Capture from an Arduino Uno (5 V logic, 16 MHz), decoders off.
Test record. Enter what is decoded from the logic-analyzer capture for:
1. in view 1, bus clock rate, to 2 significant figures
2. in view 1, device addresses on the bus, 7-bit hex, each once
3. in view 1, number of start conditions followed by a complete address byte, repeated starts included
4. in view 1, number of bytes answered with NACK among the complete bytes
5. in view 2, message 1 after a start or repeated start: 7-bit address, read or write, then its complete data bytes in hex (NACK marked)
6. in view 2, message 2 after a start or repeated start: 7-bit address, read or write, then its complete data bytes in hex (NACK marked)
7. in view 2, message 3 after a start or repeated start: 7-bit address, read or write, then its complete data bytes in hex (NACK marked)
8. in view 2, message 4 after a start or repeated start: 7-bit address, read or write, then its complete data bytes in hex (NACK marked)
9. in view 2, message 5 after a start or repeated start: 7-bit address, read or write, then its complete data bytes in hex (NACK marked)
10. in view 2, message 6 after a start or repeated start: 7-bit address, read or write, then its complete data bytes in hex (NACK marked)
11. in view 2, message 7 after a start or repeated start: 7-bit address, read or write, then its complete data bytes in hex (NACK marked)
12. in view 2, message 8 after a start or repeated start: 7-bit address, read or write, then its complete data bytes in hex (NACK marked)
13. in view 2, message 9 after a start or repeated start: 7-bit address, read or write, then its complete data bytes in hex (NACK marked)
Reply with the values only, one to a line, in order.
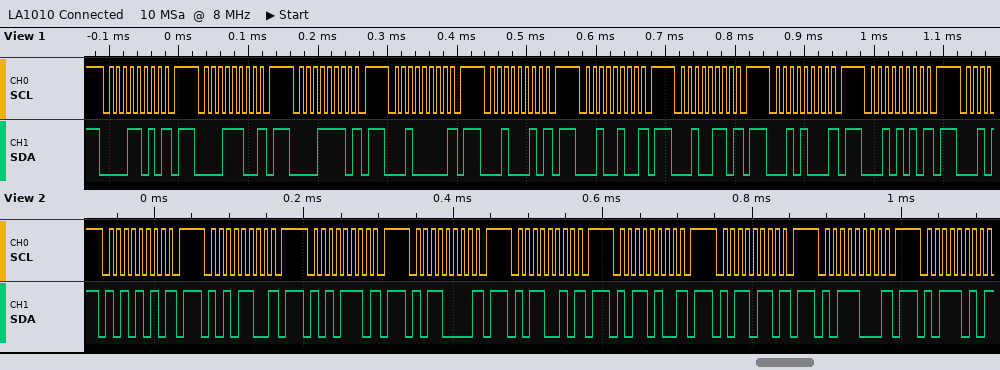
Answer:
100 kHz
0x0D 0x0E 0x0F 0x10 0x11 0x12 0x13 0x14 0x15
9
9
0x55 write NACK
0x56 write NACK
0x57 write NACK
0x58 write NACK
0x59 write NACK
0x5A write NACK
0x5B write NACK
0x5C write NACK
0x5D write NACK
